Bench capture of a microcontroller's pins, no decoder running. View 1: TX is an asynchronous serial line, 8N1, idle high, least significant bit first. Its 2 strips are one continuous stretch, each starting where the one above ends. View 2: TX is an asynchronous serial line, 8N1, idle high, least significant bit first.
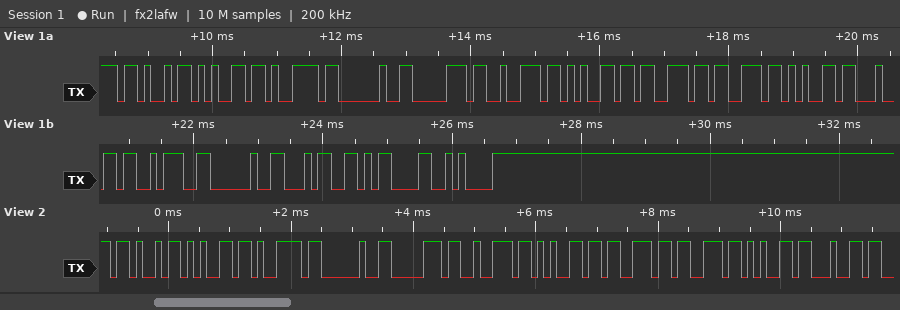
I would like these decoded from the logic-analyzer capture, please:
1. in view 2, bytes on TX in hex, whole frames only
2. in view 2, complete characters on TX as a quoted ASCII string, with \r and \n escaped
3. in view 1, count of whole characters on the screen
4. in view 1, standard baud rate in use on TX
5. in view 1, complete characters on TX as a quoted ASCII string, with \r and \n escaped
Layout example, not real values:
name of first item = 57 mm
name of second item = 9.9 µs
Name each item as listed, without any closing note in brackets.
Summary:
in view 2, bytes on TX in hex, whole frames only = 4B 65 79 20 70 72 65 73 73 65 64
in view 2, complete characters on TX as a quoted ASCII string, with \r and \n escaped = "Key pressed"
in view 1, count of whole characters on the screen = 16
in view 1, standard baud rate in use on TX = 9600 baud
in view 1, complete characters on TX as a quoted ASCII string, with \r and \n escaped = "Key pressed: 4\r\n"
